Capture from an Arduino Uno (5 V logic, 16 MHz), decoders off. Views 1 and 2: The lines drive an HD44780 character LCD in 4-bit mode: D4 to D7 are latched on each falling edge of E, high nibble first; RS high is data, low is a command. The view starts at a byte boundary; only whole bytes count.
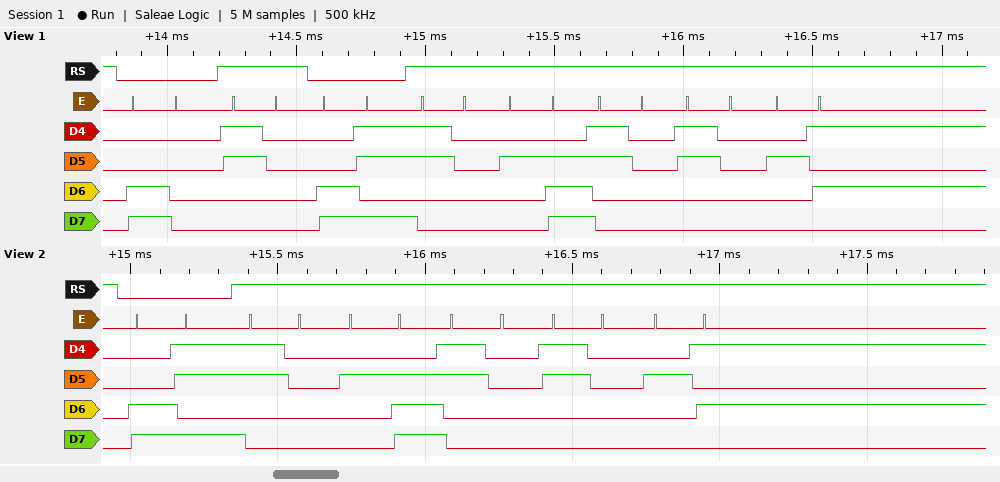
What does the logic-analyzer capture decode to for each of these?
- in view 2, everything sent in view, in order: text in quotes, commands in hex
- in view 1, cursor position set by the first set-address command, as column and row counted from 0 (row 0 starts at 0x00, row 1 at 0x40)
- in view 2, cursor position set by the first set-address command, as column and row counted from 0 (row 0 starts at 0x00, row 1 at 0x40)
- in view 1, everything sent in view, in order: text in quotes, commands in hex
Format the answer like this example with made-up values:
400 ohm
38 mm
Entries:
0xCB "0.00%"
column 0, row 1
column 11, row 1
0xC0 "0" 0xCB "0.00%"
